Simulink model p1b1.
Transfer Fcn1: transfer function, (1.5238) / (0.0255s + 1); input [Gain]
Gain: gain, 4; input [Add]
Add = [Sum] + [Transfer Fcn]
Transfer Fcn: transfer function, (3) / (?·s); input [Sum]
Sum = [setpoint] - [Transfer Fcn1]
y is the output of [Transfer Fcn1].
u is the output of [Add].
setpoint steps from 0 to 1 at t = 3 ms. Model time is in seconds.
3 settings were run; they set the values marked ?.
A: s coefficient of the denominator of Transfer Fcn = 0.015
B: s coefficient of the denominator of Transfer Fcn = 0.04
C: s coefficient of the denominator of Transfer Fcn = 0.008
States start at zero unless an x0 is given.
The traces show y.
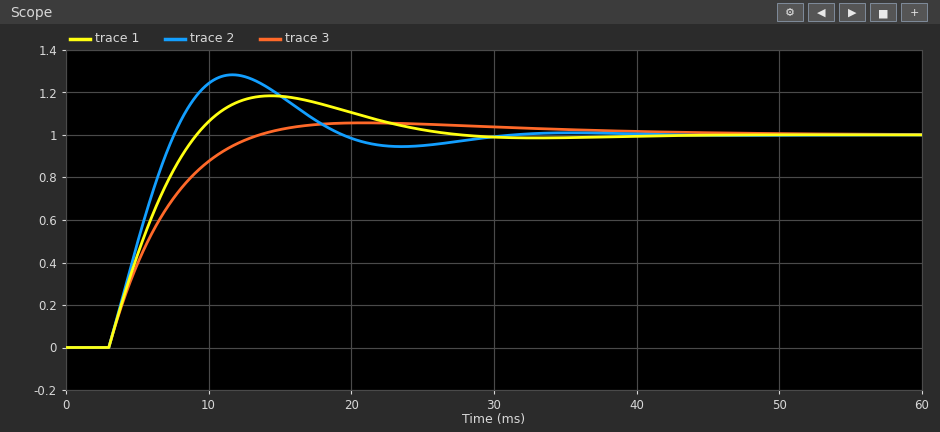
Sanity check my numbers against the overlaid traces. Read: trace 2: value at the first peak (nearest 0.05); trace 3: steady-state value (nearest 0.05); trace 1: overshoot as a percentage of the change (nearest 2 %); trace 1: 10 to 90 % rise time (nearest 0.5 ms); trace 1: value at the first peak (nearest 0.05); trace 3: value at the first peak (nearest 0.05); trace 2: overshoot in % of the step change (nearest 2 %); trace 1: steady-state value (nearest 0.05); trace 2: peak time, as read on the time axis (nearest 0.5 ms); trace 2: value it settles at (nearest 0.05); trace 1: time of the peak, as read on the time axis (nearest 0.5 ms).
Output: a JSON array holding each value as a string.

["1.30", "1.00", "18 %", "4.5 ms", "1.20", "1.05", "28 %", "1.00", "11.5 ms", "1.00", "14.5 ms"]
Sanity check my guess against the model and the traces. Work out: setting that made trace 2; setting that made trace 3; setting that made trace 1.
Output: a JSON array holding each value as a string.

["C", "B", "A"]
